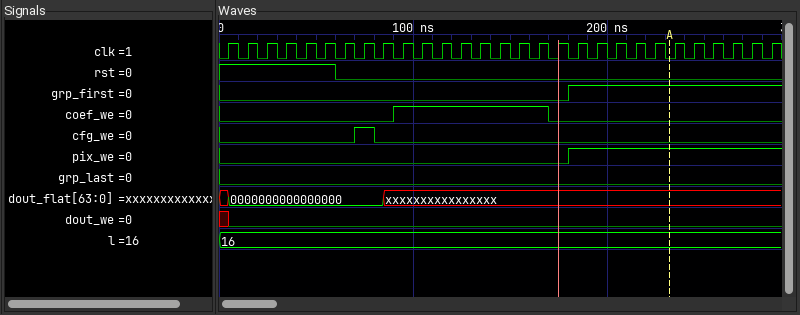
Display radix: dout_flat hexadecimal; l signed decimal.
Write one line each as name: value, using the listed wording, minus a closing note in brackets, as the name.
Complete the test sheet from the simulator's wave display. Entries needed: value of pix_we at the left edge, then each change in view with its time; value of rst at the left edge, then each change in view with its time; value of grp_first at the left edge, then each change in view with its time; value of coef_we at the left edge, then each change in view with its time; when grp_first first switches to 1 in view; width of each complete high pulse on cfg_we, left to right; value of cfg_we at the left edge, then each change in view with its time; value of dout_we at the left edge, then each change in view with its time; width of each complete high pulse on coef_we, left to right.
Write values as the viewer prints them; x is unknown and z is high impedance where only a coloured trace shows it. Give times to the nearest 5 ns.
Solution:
value of pix_we at the left edge, then each change in view with its time: 0, 1 at 180 ns
value of rst at the left edge, then each change in view with its time: 1, 0 at 60 ns
value of grp_first at the left edge, then each change in view with its time: 0, 1 at 180 ns
value of coef_we at the left edge, then each change in view with its time: 0, 1 at 90 ns, 0 at 170 ns
when grp_first first switches to 1 in view: 180 ns
width of each complete high pulse on cfg_we, left to right: 10 ns
value of cfg_we at the left edge, then each change in view with its time: 0, 1 at 70 ns, 0 at 80 ns
value of dout_we at the left edge, then each change in view with its time: x, 0 at 5 ns
width of each complete high pulse on coef_we, left to right: 80 ns
